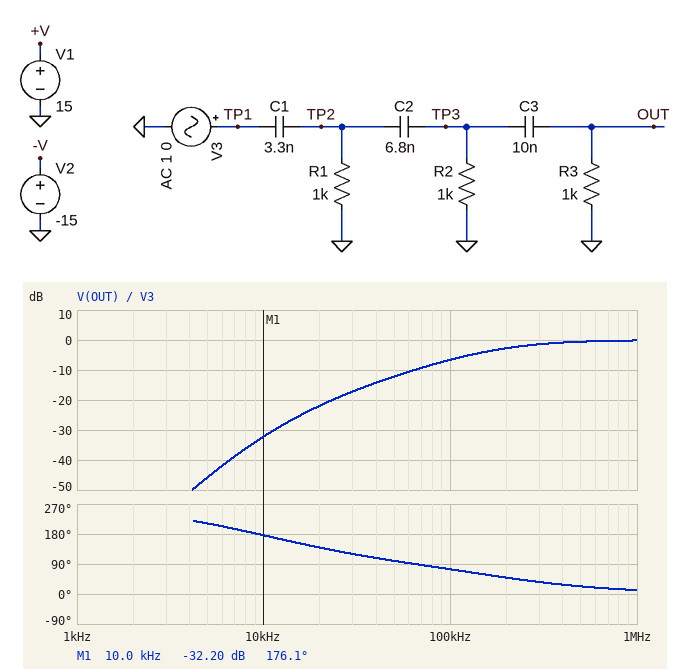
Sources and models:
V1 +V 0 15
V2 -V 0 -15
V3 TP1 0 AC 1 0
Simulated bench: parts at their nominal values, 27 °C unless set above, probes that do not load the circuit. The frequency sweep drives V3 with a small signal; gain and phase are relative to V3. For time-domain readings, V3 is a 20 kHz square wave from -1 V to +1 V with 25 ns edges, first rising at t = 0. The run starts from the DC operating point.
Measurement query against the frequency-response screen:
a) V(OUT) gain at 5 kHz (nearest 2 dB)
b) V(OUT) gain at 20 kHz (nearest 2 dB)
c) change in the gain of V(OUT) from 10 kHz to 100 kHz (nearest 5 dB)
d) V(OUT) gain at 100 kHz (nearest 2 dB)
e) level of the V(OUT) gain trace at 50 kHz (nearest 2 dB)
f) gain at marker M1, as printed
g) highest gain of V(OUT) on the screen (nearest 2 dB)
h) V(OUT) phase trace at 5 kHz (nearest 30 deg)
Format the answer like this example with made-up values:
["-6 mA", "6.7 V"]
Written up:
["-46 dB", "-22 dB", "25 dB", "-6 dB", "-12 dB", "-32.20 dB", "0 dB", "210 deg"]
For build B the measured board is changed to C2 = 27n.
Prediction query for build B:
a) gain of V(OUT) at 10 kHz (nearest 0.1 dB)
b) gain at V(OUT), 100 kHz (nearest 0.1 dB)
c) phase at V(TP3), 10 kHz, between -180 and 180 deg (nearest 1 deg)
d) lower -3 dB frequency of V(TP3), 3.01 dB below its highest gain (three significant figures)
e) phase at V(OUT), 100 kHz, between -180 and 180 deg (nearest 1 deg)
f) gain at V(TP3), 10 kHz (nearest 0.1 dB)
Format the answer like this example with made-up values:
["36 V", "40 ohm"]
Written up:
["-27.8 dB", "-5.5 dB", "91 deg", "158 kHz", "66 deg", "-22.3 dB"]
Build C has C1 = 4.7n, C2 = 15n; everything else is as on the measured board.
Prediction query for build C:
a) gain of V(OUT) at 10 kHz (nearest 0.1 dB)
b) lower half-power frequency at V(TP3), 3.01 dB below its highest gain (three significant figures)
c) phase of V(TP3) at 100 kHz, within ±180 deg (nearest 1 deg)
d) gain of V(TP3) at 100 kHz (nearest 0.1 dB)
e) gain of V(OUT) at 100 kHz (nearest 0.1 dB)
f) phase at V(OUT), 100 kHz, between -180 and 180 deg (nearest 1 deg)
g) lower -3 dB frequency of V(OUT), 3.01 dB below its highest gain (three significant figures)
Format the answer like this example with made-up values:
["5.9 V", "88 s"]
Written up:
["-26.2 dB", "122 kHz", "51 deg", "-4.0 dB", "-4.1 dB", "60 deg", "124 kHz"]
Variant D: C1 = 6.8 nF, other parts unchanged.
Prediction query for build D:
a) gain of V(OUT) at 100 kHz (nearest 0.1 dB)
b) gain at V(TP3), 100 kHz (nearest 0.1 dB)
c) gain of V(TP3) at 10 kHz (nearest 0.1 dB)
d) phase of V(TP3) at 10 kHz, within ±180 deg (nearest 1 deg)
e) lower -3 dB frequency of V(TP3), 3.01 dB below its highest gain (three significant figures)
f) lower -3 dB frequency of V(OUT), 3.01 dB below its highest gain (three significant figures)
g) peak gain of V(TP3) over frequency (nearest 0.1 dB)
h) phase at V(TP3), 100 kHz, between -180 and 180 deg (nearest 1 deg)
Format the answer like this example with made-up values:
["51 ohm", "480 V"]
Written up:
["-3.7 dB", "-3.6 dB", "-21.2 dB", "110 deg", "114 kHz", "116 kHz", "0 dB", "50 deg"]
